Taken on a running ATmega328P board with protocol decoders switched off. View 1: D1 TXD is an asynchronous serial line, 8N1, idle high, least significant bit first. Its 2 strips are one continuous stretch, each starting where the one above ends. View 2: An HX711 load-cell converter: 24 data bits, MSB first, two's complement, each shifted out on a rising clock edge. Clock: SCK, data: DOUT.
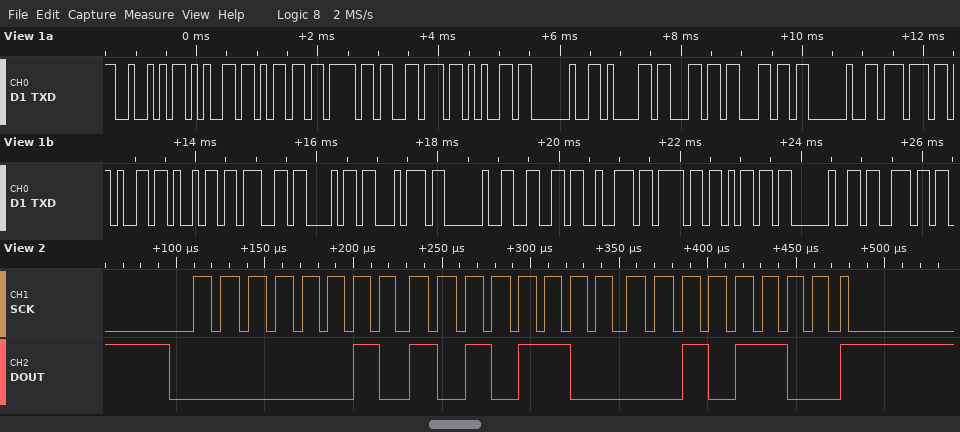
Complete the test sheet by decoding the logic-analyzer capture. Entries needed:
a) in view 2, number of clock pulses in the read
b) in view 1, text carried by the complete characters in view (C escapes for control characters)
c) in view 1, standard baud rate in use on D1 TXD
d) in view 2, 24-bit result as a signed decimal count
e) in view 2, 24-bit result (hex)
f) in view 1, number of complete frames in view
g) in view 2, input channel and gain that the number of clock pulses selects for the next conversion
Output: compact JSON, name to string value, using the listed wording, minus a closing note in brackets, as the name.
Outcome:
{"in view 2, number of clock pulses in the read": "25", "in view 1, text carried by the complete characters in view": "\"Remove all weight from s\"", "in view 1, standard baud rate in use on D1 TXD": "9600 baud", "in view 2, 24-bit result as a signed decimal count": "175148", "in view 2, 24-bit result": "0x02AC2C", "in view 1, number of complete frames in view": "24", "in view 2, input channel and gain that the number of clock pulses selects for the next conversion": "channel A, gain 128"}
